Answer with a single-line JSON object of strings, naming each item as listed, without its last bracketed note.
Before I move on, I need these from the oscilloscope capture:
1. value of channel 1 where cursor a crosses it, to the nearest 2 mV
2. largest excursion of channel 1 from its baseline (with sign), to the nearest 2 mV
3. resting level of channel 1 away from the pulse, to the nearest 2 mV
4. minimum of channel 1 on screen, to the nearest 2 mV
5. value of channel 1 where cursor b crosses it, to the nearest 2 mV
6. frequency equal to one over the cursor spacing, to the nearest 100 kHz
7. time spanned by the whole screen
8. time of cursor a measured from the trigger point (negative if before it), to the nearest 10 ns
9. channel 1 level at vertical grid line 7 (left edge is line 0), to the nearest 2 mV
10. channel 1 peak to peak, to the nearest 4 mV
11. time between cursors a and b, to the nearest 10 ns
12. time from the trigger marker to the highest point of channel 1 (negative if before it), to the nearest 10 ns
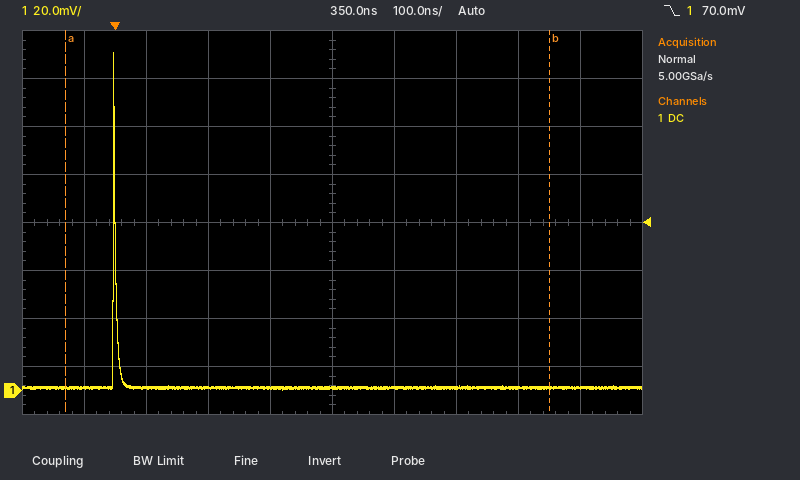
{"value of channel 1 where cursor a crosses it, to the nearest 2 mV": "2 mV", "largest excursion of channel 1 from its baseline (with sign), to the nearest 2 mV": "+140 mV", "resting level of channel 1 away from the pulse, to the nearest 2 mV": "2 mV", "minimum of channel 1 on screen, to the nearest 2 mV": "0 mV", "value of channel 1 where cursor b crosses it, to the nearest 2 mV": "2 mV", "frequency equal to one over the cursor spacing, to the nearest 100 kHz": "1.3 MHz", "time spanned by the whole screen": "1 µs", "time of cursor a measured from the trigger point (negative if before it), to the nearest 10 ns": "-80 ns", "channel 1 level at vertical grid line 7 (left edge is line 0), to the nearest 2 mV": "2 mV", "channel 1 peak to peak, to the nearest 4 mV": "140 mV", "time between cursors a and b, to the nearest 10 ns": "780 ns", "time from the trigger marker to the highest point of channel 1 (negative if before it), to the nearest 10 ns": "0 ns"}
